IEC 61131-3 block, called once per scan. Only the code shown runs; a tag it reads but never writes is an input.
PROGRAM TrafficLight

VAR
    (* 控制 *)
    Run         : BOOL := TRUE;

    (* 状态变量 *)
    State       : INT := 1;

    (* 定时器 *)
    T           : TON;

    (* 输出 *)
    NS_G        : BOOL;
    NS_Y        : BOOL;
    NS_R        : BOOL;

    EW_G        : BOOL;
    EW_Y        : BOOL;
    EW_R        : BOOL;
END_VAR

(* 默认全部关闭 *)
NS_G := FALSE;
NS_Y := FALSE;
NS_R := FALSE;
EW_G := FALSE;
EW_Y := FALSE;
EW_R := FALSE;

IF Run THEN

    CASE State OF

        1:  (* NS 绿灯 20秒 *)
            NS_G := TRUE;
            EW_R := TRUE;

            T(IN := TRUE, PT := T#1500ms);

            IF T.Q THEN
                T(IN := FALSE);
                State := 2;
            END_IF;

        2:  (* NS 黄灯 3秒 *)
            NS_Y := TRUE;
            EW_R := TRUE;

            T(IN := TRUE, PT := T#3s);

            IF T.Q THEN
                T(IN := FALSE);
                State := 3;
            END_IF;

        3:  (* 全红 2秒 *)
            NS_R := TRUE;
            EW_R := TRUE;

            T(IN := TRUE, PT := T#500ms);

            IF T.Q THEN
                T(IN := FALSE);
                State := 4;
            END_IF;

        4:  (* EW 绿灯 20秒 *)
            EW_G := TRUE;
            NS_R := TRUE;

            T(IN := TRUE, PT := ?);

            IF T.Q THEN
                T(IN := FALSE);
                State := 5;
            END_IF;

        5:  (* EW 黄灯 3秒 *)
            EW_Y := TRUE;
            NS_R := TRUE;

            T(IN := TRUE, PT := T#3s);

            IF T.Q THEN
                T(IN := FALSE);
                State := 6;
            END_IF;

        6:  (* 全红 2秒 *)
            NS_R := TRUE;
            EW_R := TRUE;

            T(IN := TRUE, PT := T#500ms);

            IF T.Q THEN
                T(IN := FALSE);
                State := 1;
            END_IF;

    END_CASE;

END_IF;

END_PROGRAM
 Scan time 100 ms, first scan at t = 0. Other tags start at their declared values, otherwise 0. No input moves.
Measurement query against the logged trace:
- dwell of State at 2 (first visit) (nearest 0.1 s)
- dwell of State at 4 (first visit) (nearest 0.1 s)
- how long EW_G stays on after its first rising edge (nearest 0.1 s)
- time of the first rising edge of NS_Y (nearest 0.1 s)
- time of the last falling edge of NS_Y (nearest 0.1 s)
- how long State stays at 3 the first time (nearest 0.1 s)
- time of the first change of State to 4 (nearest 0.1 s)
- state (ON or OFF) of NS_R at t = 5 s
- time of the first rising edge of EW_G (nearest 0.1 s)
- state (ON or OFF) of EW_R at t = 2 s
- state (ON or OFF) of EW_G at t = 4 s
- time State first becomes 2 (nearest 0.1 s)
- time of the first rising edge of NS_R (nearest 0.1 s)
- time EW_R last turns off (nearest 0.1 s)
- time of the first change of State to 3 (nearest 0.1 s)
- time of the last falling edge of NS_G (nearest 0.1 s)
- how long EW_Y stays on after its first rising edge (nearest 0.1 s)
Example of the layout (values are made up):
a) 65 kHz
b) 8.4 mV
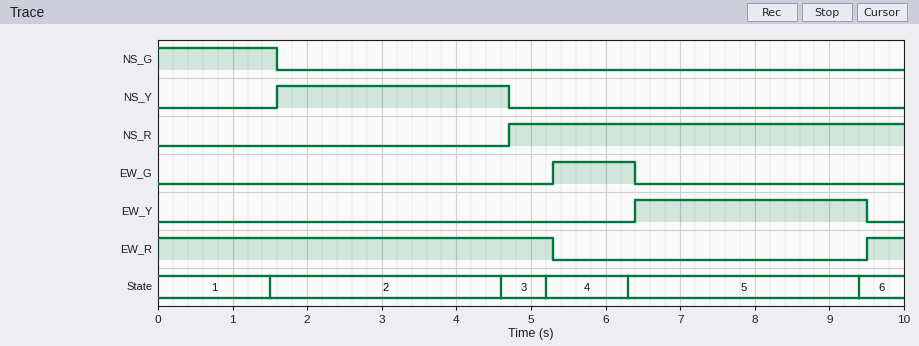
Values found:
a) 3.1 s
b) 1.1 s
c) 1.1 s
d) 1.6 s
e) 4.7 s
f) 0.6 s
g) 5.2 s
h) ON
i) 5.3 s
j) ON
k) OFF
l) 1.5 s
m) 4.7 s
n) 5.3 s
o) 4.6 s
p) 1.6 s
q) 3.1 s
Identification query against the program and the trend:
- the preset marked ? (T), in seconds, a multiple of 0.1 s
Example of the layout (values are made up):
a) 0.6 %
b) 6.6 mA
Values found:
a) 1.0 s
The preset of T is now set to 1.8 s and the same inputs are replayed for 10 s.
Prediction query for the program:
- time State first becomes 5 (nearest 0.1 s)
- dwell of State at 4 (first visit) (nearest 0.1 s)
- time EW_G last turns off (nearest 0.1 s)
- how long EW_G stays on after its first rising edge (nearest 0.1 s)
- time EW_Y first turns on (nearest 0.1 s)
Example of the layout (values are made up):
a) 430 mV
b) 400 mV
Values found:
a) 7.1 s
b) 1.9 s
c) 7.2 s
d) 1.9 s
e) 7.2 s
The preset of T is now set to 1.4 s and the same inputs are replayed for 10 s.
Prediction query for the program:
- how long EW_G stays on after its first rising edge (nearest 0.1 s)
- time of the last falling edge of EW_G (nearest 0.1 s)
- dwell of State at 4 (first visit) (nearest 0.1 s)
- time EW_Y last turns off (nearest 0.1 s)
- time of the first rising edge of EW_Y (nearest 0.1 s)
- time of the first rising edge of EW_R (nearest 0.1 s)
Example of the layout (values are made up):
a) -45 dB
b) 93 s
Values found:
a) 1.5 s
b) 6.8 s
c) 1.5 s
d) 9.9 s
e) 6.8 s
f) 9.9 s
